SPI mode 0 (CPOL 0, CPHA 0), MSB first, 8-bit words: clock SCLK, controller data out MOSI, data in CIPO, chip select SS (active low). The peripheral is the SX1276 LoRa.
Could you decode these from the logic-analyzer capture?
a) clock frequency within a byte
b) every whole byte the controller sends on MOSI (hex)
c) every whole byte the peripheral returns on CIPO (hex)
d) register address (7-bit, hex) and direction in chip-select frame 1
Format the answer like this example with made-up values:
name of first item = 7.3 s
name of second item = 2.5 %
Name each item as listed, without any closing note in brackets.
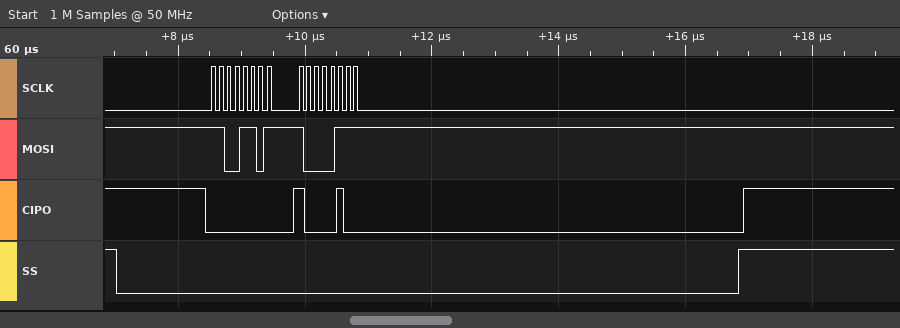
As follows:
clock frequency within a byte = 8 MHz
every whole byte the controller sends on MOSI = CD 87
every whole byte the peripheral returns on CIPO = 00 84
register address (7-bit, hex) and direction in chip-select frame 1 = 0x4D write
